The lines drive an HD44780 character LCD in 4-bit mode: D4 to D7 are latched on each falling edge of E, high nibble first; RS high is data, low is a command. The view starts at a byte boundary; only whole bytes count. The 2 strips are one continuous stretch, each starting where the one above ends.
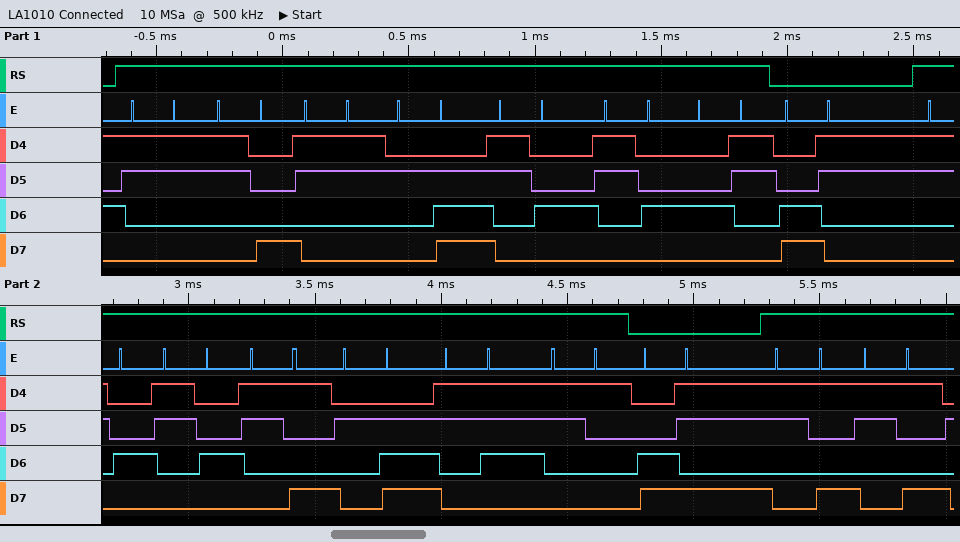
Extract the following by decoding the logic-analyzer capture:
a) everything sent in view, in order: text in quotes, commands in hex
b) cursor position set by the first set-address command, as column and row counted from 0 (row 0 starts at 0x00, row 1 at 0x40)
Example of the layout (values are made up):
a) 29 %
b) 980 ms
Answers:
a) "383.44C" 0xC3 "449.71" 0xCB "99"
b) column 3, row 1
